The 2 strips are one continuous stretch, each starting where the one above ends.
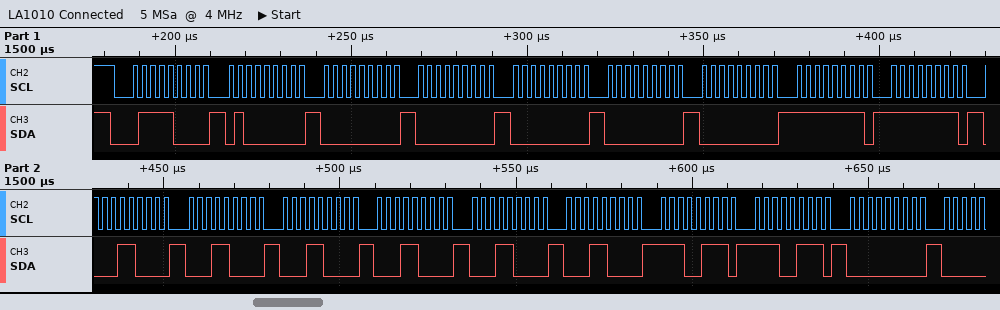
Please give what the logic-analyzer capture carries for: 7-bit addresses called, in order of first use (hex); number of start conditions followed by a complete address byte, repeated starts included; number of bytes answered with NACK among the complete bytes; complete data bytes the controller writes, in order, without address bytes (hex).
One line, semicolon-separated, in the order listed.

0x3C; 1; 0; 40 00 00 00 00 00 FF FF 18 18 18 18 18 18 E7 E7 00
